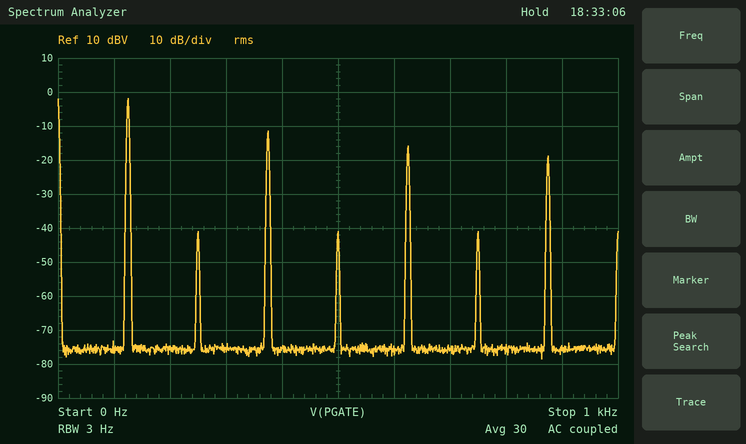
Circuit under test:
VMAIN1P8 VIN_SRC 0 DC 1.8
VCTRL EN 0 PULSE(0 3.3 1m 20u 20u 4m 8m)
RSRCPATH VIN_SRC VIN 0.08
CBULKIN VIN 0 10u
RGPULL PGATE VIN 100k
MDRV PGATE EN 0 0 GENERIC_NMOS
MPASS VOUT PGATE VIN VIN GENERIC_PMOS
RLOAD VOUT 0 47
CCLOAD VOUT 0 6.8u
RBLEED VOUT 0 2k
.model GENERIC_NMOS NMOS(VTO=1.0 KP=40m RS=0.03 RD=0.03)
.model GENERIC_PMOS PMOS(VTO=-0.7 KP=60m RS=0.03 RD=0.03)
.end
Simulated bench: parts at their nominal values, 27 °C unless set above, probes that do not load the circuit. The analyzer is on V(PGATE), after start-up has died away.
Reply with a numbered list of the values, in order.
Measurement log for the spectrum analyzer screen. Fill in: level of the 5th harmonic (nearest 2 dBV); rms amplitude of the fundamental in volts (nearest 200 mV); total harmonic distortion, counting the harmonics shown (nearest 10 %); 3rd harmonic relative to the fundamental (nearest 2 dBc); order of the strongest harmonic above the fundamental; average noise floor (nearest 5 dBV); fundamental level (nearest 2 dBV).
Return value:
1. -16 dBV
2. 800 mV
3. 40 %
4. -10 dBc
5. 3
6. -75 dBV
7. -2 dBV
